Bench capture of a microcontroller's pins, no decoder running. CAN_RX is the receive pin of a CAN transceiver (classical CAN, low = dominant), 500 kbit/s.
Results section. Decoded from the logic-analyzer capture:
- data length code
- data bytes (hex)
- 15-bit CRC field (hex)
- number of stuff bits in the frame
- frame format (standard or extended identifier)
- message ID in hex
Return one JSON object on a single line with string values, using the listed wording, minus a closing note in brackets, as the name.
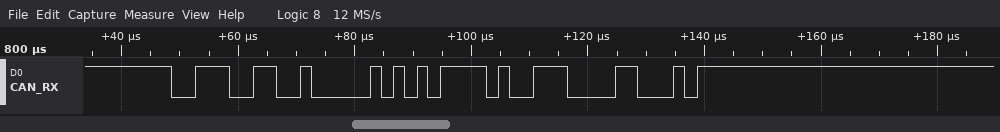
{"data length code": "1", "data bytes": "5E", "15-bit CRC field": "0x4E18", "number of stuff bits in the frame": "1", "frame format": "standard", "message ID in hex": "0x399"}
